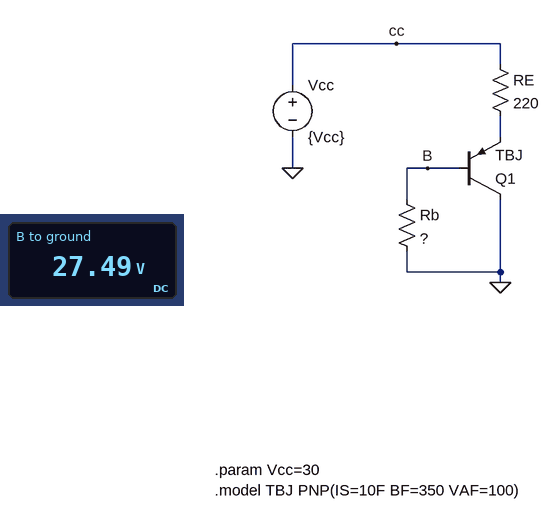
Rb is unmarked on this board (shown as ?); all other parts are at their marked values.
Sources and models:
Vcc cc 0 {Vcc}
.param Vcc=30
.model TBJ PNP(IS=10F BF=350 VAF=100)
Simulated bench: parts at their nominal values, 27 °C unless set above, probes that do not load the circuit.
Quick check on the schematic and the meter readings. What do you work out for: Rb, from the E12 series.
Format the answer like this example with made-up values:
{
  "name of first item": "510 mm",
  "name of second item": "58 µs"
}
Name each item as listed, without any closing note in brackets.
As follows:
{
  "Rb, from the E12 series": "1.5 MΩ"
}
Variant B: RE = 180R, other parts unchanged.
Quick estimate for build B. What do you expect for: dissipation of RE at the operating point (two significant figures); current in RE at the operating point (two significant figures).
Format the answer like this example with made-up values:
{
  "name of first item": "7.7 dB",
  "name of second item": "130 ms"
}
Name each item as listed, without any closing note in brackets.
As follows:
{
  "dissipation of RE at the operating point": "12 mW",
  "current in RE at the operating point": "8.3 mA"
}
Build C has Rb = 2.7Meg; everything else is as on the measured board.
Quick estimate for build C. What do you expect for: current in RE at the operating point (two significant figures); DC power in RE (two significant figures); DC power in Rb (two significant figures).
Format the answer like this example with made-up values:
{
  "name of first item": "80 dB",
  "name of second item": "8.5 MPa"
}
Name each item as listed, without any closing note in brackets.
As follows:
{
  "current in RE at the operating point": "4.7 mA",
  "DC power in RE": "4.9 mW",
  "DC power in Rb": "300 µW"
}
